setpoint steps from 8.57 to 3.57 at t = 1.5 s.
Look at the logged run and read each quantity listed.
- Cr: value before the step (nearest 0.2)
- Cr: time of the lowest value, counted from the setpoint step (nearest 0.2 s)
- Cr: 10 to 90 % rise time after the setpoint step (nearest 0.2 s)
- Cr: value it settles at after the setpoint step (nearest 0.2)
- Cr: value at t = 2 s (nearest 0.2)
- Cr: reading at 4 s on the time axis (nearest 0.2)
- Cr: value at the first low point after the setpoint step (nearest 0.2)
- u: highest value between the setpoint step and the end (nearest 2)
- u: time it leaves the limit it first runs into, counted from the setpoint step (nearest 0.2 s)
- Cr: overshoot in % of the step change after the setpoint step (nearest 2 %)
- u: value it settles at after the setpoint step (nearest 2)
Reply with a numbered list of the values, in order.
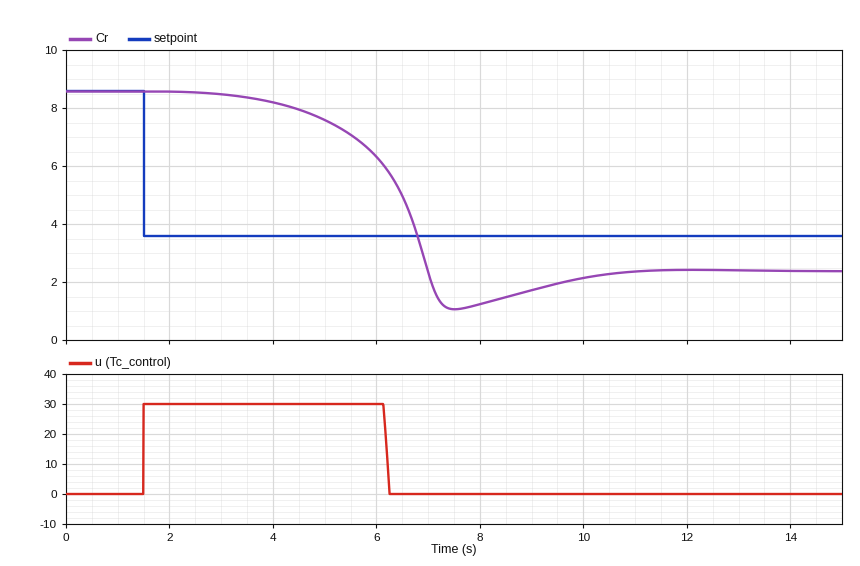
1. 8.6
2. 6.0 s
3. 2.4 s
4. 2.4
5. 8.6
6. 8.2
7. 1.0
8. 30
9. 4.6 s
10. 22 %
11. 0
